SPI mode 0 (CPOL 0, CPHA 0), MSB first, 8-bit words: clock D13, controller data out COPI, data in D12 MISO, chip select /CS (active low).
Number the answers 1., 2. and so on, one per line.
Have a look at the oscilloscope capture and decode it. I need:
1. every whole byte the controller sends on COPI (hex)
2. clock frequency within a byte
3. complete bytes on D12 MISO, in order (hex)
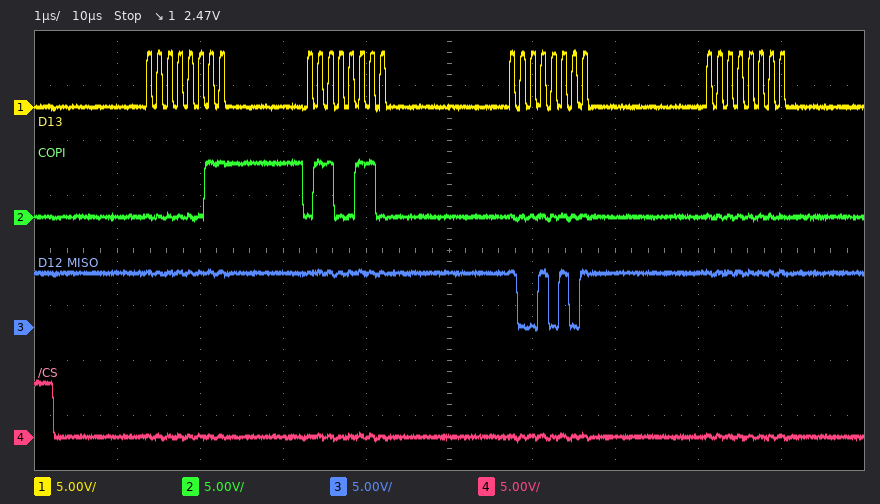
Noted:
1. 03 66 00 00
2. 8 MHz
3. FF FF 95 FF
